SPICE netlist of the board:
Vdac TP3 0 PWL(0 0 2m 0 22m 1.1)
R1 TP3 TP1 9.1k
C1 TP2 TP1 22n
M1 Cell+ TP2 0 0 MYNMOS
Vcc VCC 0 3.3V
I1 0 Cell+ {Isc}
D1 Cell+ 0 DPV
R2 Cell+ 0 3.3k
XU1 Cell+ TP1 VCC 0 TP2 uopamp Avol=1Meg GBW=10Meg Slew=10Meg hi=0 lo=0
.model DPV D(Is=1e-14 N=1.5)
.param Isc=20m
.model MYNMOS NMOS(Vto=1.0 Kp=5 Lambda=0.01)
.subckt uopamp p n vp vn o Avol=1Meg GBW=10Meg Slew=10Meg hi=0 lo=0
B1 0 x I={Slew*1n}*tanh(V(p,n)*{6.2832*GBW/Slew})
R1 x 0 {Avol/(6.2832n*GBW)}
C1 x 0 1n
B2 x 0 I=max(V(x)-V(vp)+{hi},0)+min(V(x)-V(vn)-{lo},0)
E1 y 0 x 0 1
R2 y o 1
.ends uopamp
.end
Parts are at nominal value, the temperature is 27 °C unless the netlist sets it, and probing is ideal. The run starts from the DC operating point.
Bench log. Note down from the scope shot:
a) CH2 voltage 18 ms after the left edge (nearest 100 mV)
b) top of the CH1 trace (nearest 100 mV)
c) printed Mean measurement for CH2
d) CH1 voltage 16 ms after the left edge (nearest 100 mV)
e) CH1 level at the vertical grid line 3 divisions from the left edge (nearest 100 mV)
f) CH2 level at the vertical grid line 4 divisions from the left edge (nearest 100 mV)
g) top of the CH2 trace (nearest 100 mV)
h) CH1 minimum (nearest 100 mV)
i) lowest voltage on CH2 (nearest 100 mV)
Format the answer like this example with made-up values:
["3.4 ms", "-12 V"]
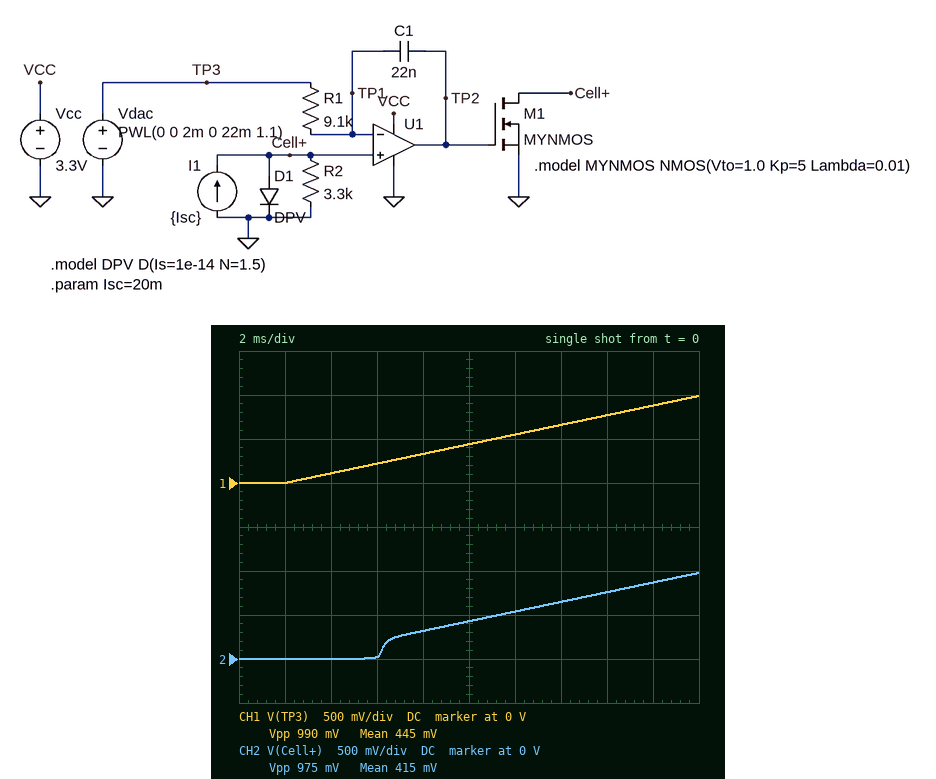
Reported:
["900 mV", "1.0 V", "415 mV", "800 mV", "200 mV", "300 mV", "1.0 V", "0 V", "0 V"]
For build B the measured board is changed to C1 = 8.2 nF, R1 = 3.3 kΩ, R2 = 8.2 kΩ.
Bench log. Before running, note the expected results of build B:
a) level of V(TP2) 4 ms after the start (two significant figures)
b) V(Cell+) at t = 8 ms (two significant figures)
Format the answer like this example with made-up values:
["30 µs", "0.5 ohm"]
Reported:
["1.1 V", "330 mV"]
